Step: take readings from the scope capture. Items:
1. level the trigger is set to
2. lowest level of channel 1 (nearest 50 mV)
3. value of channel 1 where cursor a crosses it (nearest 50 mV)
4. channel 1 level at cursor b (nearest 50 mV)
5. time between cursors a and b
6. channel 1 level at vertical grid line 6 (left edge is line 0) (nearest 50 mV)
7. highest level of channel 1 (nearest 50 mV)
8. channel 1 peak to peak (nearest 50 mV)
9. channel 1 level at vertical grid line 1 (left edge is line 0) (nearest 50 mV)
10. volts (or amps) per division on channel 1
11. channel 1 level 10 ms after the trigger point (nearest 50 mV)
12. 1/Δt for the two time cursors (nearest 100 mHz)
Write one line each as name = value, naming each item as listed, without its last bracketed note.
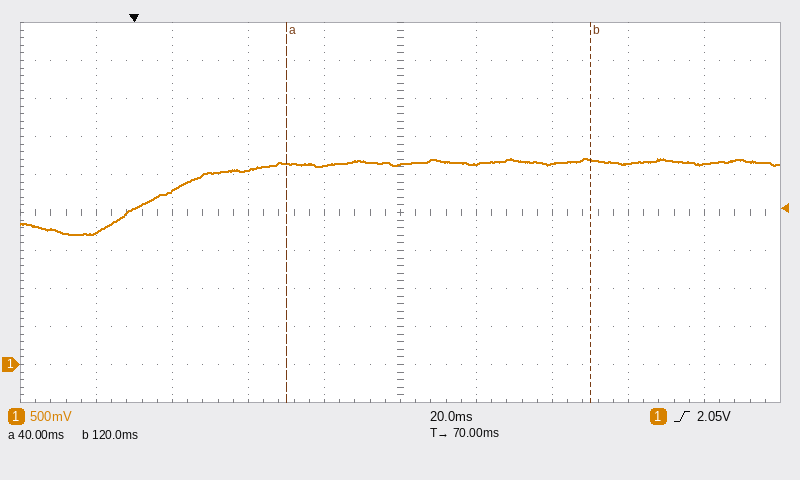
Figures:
level the trigger is set to = 2.05 V
lowest level of channel 1 = 1.70 V
value of channel 1 where cursor a crosses it = 2.65 V
channel 1 level at cursor b = 2.70 V
time between cursors a and b = 80 ms
channel 1 level at vertical grid line 6 (left edge is line 0) = 2.65 V
highest level of channel 1 = 2.70 V
channel 1 peak to peak = 1.00 V
channel 1 level at vertical grid line 1 (left edge is line 0) = 1.75 V
volts (or amps) per division on channel 1 = 500 mV
channel 1 level 10 ms after the trigger point = 2.30 V
1/Δt for the two time cursors = 12.5 Hz
